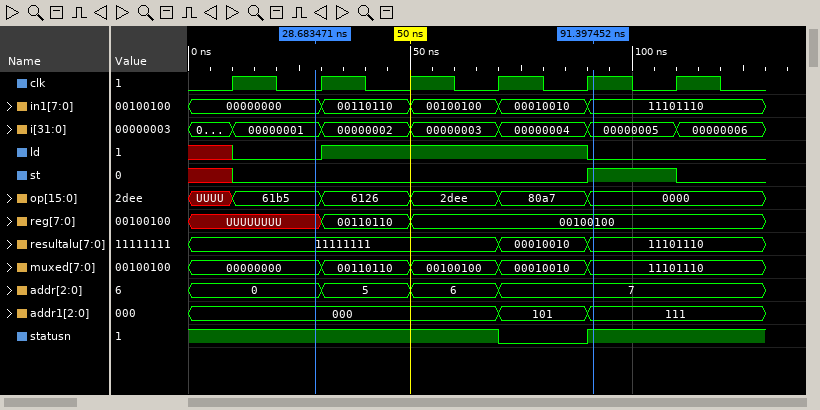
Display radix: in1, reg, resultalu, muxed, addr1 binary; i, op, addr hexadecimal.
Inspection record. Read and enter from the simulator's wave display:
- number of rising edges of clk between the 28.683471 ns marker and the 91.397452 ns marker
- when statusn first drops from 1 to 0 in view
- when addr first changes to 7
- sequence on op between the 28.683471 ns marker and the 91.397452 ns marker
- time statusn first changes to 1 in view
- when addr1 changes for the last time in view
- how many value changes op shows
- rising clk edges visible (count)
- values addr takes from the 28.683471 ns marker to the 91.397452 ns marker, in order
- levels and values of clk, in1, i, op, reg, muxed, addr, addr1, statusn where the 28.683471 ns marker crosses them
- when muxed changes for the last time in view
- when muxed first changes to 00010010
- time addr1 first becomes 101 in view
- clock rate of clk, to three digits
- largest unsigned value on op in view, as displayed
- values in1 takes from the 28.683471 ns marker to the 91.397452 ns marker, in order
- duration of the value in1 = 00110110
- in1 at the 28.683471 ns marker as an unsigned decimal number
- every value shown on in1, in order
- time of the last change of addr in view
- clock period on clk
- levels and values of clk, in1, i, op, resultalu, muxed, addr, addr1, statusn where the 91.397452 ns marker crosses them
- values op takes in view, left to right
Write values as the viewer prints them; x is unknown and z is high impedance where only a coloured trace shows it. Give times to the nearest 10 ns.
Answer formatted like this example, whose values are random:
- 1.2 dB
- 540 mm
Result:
- 4
- 70 ns
- 70 ns
- 61b5, 6126, 2dee, 80a7, 0000
- 90 ns
- 90 ns
- 5
- 6
- 0, 5, 6, 7
- clk=0, in1=00000000, i=00000001, op=61b5, reg=UUUUUUUU, muxed=00000000, addr=0, addr1=000, statusn=1
- 90 ns
- 70 ns
- 70 ns
- 50.0 MHz
- 80a7
- 00000000, 00110110, 00100100, 00010010, 11101110
- 20 ns
- 0
- 00000000, 00110110, 00100100, 00010010, 11101110
- 70 ns
- 20 ns
- clk=1, in1=11101110, i=00000005, op=0000, resultalu=11101110, muxed=11101110, addr=7, addr1=111, statusn=1
- UUUU, 61b5, 6126, 2dee, 80a7, 0000
